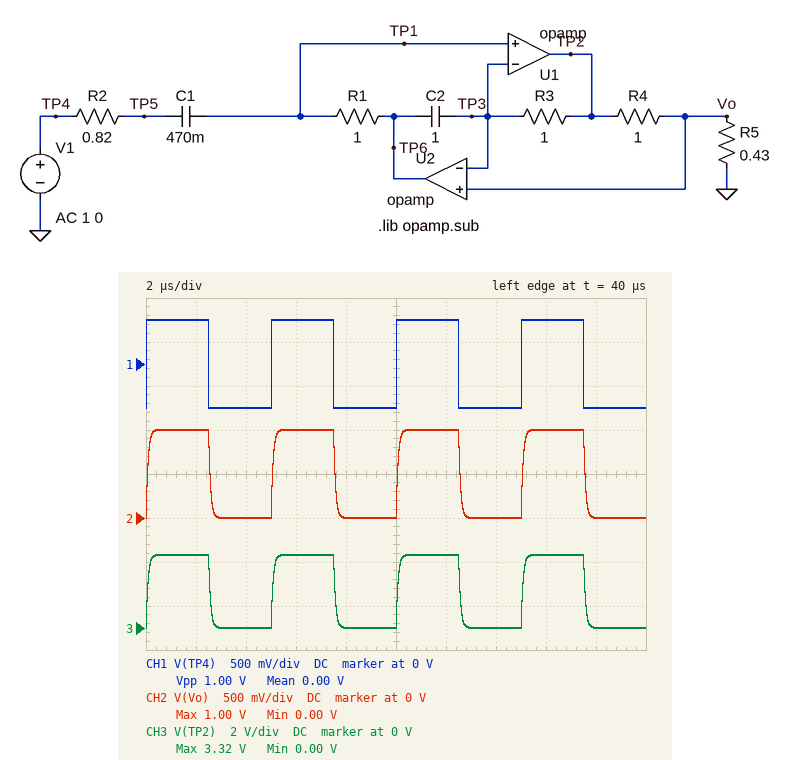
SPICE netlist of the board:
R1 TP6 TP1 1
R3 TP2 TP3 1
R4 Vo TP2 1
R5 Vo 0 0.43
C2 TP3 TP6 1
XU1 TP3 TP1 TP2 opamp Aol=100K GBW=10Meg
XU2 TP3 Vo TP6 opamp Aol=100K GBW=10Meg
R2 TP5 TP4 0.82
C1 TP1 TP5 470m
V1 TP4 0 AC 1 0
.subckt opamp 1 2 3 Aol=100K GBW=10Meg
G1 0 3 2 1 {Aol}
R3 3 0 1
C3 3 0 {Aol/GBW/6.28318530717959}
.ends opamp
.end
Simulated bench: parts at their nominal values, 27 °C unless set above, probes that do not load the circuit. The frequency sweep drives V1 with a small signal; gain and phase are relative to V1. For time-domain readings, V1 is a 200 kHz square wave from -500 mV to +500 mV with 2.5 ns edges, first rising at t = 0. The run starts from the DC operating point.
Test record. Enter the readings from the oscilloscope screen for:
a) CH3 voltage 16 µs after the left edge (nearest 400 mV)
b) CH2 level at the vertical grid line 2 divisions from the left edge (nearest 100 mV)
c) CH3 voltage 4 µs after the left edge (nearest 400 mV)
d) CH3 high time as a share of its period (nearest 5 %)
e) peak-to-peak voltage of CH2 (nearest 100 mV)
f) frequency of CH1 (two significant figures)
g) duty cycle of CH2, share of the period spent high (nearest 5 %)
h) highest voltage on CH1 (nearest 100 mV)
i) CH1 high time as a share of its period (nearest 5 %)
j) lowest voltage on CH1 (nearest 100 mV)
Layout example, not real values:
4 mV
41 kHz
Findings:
3.2 V
0 V
0 V
50 %
1.0 V
200 kHz
50 %
500 mV
50 %
-500 mV
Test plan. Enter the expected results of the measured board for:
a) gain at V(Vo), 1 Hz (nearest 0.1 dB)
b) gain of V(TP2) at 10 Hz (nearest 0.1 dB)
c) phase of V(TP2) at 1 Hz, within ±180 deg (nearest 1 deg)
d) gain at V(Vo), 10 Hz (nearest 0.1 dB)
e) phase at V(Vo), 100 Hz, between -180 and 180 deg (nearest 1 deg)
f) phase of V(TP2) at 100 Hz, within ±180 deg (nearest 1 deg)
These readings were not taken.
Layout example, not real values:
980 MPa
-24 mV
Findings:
0.7 dB
10.4 dB
19 deg
0 dB
0 deg
0 deg
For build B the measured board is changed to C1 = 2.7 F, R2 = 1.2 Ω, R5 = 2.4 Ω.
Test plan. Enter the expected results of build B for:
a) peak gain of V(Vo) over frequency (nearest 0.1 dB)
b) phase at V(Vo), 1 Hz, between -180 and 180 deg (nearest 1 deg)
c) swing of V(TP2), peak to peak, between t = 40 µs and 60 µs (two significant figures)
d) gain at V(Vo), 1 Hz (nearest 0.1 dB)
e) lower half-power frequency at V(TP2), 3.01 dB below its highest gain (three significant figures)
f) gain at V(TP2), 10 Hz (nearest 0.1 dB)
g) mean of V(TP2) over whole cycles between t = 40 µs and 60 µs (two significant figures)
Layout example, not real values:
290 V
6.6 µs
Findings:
0.2 dB
5 deg
1.4 V
0 dB
57.8 mHz
3.0 dB
710 mV
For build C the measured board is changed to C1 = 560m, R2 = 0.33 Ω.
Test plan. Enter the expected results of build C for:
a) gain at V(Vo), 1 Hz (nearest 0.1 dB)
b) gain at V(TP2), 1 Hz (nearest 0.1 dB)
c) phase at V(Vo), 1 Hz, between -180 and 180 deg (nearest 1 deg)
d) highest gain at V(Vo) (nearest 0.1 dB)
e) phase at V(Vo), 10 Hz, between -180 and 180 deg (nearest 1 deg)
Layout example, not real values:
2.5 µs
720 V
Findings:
0.9 dB
11.3 dB
8 deg
8.6 dB
1 deg
